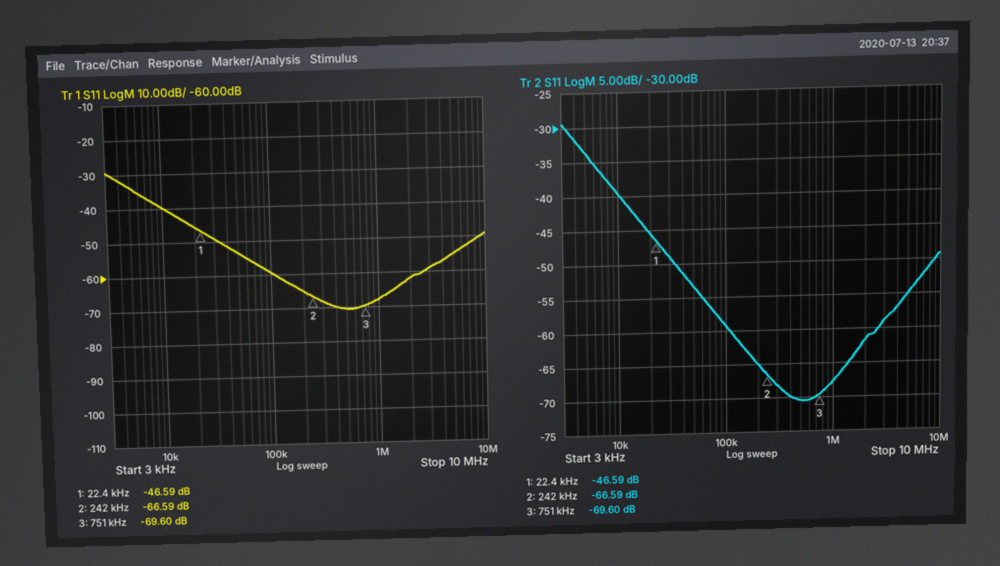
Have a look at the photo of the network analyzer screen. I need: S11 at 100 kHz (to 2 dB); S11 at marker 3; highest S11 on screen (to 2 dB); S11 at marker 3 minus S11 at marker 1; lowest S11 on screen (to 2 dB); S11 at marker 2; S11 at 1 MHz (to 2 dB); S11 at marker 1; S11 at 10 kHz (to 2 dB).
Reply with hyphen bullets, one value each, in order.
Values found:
- -60 dB
- -69.60 dB
- -30 dB
- -23.01 dB
- -70 dB
- -66.59 dB
- -68 dB
- -46.59 dB
- -40 dB
